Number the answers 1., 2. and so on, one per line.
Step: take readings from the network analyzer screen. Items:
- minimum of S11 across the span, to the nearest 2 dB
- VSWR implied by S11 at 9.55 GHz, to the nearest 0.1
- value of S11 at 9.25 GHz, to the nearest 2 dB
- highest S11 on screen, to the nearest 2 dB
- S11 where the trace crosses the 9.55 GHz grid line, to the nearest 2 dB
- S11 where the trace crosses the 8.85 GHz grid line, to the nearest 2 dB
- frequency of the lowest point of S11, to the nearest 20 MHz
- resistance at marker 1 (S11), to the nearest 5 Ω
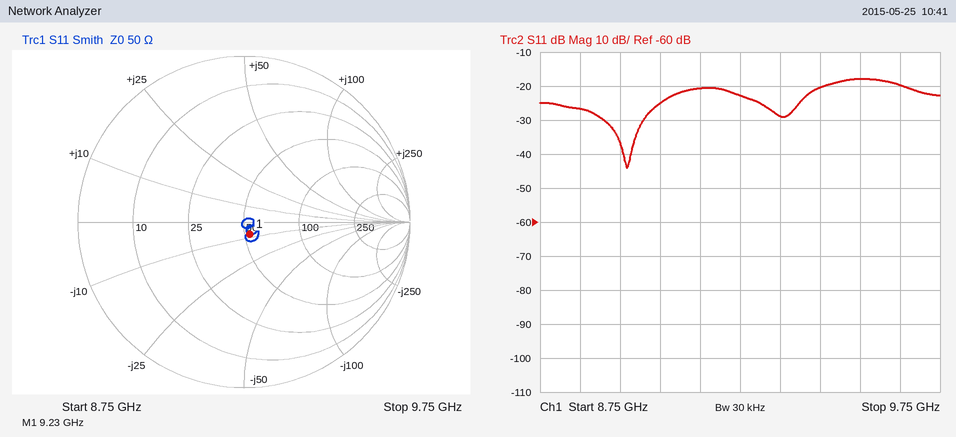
1. -44 dB
2. 1.3
3. -22 dB
4. -18 dB
5. -18 dB
6. -26 dB
7. 8.96 GHz
8. 55 Ω
